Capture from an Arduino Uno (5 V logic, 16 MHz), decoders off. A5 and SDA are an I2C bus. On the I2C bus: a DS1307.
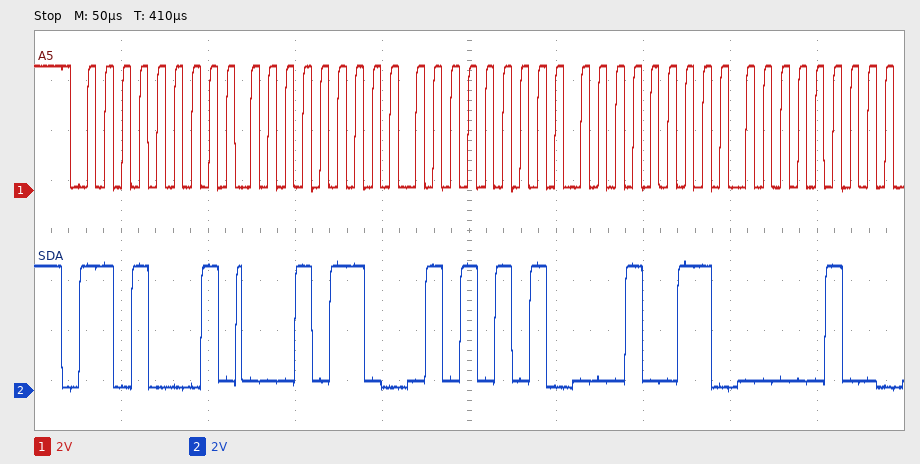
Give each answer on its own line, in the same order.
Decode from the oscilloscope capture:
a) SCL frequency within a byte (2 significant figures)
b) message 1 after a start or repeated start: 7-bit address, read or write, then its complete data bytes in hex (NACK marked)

100 kHz
0x68 read: 16 55 13 04
